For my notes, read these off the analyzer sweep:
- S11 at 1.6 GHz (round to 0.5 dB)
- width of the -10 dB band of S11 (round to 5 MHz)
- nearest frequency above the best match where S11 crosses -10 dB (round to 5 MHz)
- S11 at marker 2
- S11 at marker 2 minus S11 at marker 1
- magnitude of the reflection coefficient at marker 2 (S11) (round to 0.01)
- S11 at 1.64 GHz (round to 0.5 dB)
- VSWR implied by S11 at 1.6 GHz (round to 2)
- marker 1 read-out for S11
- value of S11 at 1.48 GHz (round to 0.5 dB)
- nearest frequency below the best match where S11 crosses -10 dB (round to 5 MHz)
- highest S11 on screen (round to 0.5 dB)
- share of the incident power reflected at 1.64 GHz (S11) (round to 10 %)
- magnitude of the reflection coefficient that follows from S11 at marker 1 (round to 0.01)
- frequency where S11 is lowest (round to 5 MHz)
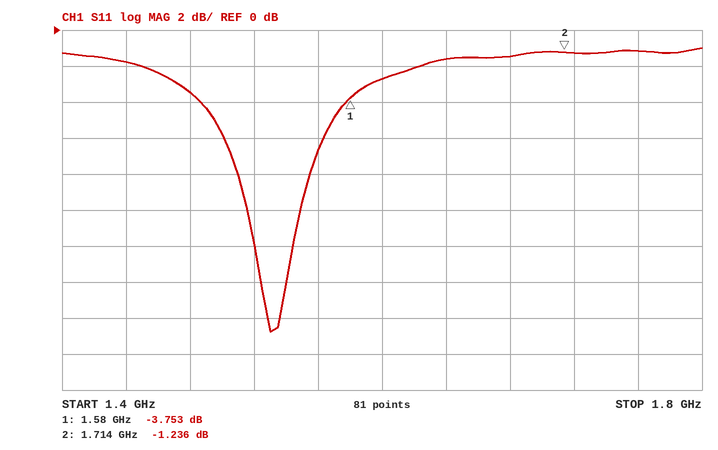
-2.5 dB
35 MHz
1.550 GHz
-1.236 dB
2.517 dB
0.87
-1.5 dB
6
-3.753 dB
-3.5 dB
1.515 GHz
-1.0 dB
70 %
0.65
1.530 GHz
